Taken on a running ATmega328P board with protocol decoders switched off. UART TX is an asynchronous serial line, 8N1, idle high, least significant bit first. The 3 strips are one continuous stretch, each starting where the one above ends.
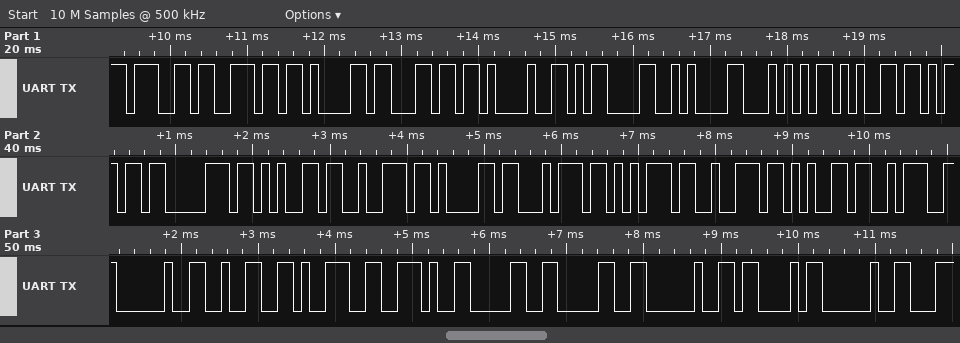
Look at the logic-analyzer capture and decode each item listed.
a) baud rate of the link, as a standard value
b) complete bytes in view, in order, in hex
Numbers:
9600 baud
0x67 0x6E 0x61 0x6C 0x21 0x0D 0x0A 0x54 0x65 0x6D 0x70 0x65 0x72 0x61 0x74 0x75 0x72 0x65 0x3A 0x20 0x32 0x39 0x2E 0x30 0x30 0x20 0x43 0x20
